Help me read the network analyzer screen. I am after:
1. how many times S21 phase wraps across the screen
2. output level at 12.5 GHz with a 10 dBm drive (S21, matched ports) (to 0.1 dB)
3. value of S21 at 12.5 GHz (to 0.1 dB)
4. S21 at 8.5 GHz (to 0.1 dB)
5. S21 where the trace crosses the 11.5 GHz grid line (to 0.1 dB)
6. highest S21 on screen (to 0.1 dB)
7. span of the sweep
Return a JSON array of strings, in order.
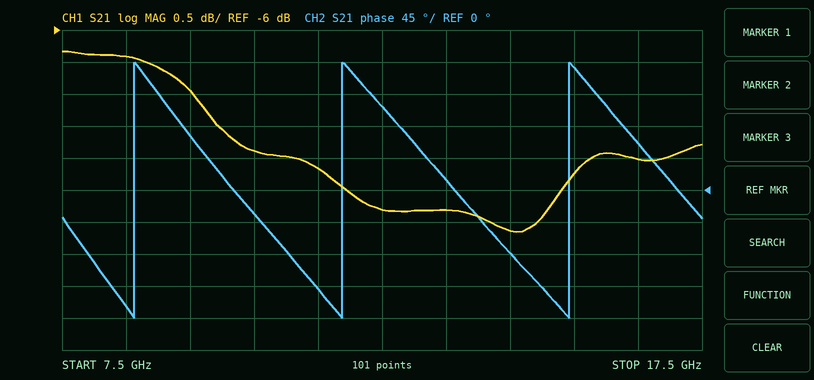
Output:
["3", "1.2 dBm", "-8.8 dB", "-6.4 dB", "-8.2 dB", "-6.3 dB", "10 GHz"]
